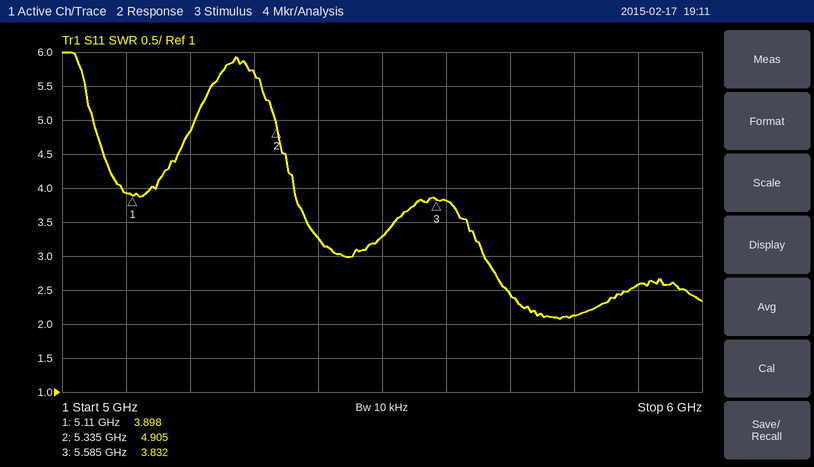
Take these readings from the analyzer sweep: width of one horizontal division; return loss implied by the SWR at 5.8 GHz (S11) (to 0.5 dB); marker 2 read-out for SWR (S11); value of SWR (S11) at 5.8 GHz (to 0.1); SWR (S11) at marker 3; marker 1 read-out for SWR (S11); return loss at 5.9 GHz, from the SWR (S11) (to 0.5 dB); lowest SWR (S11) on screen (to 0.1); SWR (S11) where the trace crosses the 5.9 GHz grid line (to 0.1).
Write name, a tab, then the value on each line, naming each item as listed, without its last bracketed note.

width of one horizontal division	100 MHz
return loss implied by the SWR at 5.8 GHz (S11)	9.0 dB
marker 2 read-out for SWR	4.905
value of SWR (S11) at 5.8 GHz	2.1
SWR (S11) at marker 3	3.832
marker 1 read-out for SWR	3.898
return loss at 5.9 GHz, from the SWR (S11)	7.0 dB
lowest SWR (S11) on screen	2.1
SWR (S11) where the trace crosses the 5.9 GHz grid line	2.6
